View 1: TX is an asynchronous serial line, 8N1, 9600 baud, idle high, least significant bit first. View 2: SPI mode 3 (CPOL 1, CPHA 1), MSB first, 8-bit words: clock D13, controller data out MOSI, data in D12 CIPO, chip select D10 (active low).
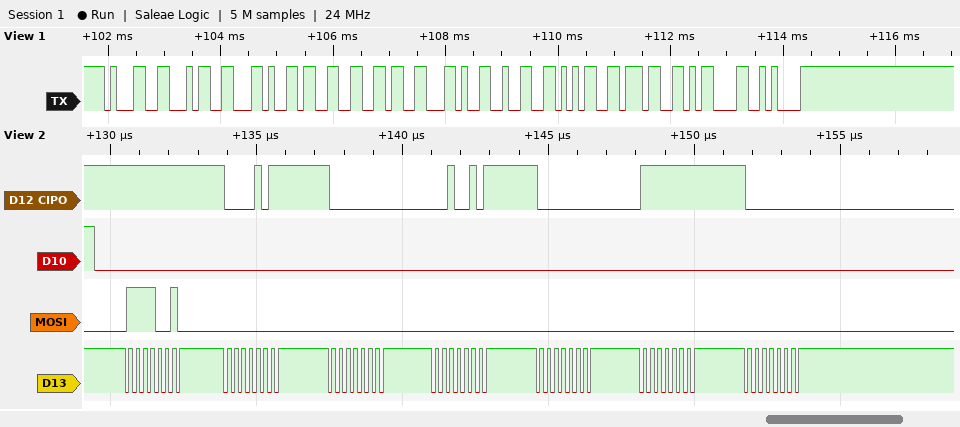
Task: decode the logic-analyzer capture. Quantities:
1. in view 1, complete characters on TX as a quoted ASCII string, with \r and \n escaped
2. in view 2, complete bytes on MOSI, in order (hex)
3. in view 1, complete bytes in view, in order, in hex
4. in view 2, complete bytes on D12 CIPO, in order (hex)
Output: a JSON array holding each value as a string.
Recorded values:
["\"14,36,257\\r\\n\"", "F2 00 00 00 00 00 00", "0x31 0x34 0x2C 0x33 0x36 0x2C 0x32 0x35 0x37 0x0D 0x0A", "FF 0B 00 25 00 FF 00"]
